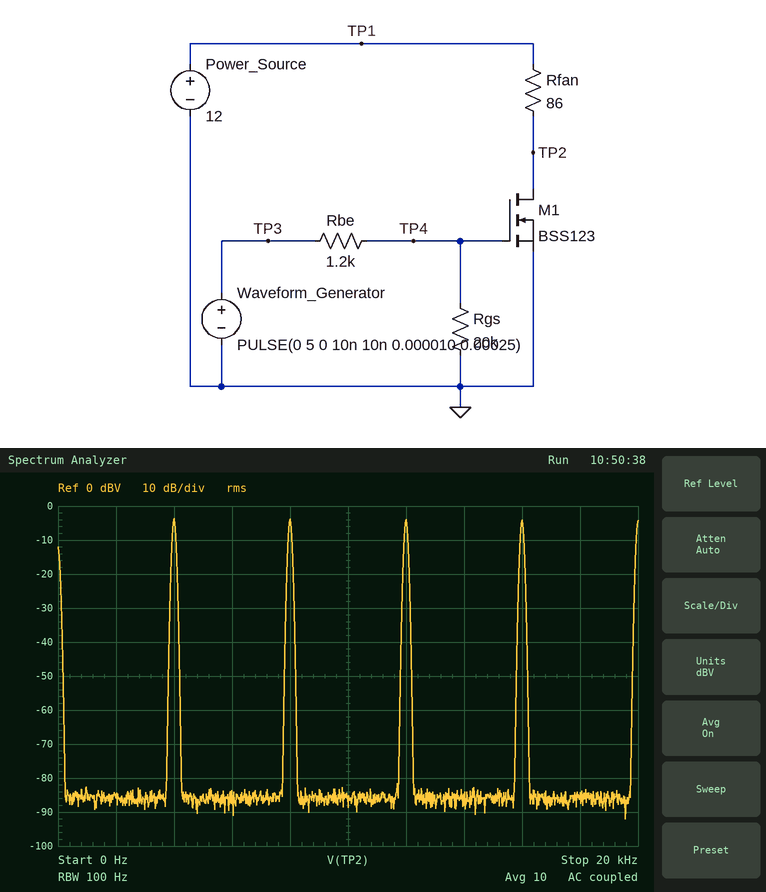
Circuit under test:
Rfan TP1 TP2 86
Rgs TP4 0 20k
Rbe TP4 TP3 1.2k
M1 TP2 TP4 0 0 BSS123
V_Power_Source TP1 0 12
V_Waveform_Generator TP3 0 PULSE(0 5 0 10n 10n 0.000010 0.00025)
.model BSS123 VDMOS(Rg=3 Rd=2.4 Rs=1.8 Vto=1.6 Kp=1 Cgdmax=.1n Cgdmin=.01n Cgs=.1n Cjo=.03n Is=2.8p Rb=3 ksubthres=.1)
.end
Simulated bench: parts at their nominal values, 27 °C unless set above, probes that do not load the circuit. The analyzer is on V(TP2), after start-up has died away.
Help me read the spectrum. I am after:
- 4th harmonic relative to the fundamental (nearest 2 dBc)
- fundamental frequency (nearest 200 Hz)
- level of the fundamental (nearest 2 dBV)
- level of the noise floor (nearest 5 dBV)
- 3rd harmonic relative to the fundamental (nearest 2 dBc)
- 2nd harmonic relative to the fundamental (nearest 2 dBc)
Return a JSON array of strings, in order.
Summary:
["0 dBc", "4.0 kHz", "-4 dBV", "-85 dBV", "0 dBc", "0 dBc"]
